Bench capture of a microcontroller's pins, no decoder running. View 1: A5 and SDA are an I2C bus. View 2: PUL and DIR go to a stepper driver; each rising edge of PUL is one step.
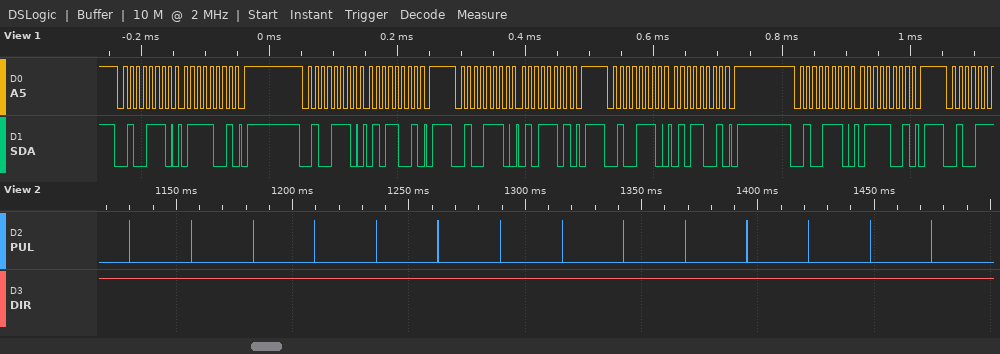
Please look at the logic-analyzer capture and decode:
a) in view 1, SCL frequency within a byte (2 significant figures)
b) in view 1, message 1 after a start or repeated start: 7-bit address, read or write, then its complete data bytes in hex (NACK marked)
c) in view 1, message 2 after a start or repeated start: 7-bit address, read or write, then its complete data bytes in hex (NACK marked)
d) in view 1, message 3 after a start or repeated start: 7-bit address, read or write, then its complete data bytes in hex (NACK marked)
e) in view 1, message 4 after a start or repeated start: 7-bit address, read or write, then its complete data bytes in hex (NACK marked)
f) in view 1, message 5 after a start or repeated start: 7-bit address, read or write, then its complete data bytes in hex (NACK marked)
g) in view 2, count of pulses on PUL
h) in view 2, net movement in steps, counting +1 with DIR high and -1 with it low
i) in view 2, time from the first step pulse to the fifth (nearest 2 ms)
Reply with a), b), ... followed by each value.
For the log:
a) 100 kHz
b) 0x27 write: 79
c) 0x27 write: 59
d) 0x27 write: 5D
e) 0x27 write: 59
f) 0x27 write: 79
g) 14
h) +14
i) 106 ms
